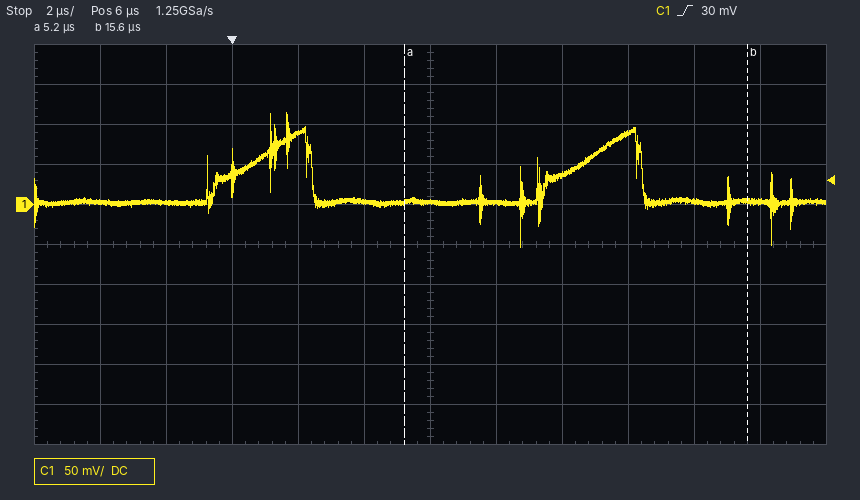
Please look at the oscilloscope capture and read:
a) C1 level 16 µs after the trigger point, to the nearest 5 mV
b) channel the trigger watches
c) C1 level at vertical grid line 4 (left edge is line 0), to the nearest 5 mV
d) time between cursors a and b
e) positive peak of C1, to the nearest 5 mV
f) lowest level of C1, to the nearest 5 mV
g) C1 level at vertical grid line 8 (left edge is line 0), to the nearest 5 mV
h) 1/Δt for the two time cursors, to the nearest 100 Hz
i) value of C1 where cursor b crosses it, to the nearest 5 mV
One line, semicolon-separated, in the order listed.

5 mV; C1; 90 mV; 10.4 µs; 115 mV; -55 mV; 35 mV; 96.2 kHz; 5 mV
